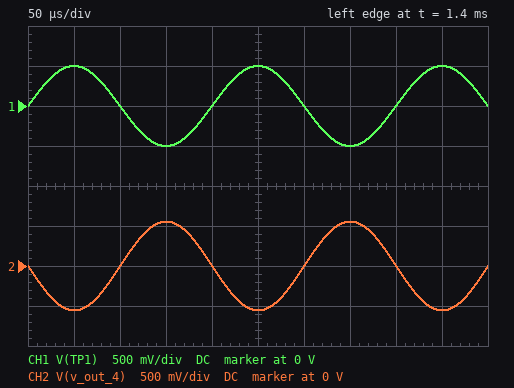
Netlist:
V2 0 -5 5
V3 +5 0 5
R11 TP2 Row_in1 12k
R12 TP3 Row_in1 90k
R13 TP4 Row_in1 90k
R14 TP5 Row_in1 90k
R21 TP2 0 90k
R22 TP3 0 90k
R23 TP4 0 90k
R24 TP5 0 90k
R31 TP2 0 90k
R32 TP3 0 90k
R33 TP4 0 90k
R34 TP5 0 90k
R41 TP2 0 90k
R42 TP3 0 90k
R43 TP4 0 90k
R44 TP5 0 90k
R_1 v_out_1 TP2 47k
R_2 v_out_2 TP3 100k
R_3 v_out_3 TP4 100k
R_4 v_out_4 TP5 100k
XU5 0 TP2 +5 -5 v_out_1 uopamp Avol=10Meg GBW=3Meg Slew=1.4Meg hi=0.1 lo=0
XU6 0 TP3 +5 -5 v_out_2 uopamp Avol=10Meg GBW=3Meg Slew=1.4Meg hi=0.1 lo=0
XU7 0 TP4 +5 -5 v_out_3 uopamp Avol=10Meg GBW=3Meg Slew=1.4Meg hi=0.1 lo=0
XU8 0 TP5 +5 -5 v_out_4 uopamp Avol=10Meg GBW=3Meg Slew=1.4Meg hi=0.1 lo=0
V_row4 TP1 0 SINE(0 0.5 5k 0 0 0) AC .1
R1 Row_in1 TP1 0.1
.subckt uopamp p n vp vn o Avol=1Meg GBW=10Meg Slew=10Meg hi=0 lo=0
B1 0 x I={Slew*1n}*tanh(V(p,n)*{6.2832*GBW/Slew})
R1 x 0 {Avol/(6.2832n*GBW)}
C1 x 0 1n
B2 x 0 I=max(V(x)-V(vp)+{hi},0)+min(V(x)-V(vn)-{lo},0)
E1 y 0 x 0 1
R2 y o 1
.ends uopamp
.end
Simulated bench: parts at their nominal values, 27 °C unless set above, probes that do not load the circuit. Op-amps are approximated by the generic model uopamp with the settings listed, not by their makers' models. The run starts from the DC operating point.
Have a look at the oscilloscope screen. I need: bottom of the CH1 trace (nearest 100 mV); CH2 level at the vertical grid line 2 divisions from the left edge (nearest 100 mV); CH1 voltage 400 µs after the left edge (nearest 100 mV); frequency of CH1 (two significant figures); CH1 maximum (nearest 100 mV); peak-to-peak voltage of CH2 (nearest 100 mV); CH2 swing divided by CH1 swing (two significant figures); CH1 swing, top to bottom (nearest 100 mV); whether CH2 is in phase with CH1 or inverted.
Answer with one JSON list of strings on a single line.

["-500 mV", "0 V", "0 V", "5.0 kHz", "500 mV", "1.1 V", "1.1", "1.0 V", "inverted"]
